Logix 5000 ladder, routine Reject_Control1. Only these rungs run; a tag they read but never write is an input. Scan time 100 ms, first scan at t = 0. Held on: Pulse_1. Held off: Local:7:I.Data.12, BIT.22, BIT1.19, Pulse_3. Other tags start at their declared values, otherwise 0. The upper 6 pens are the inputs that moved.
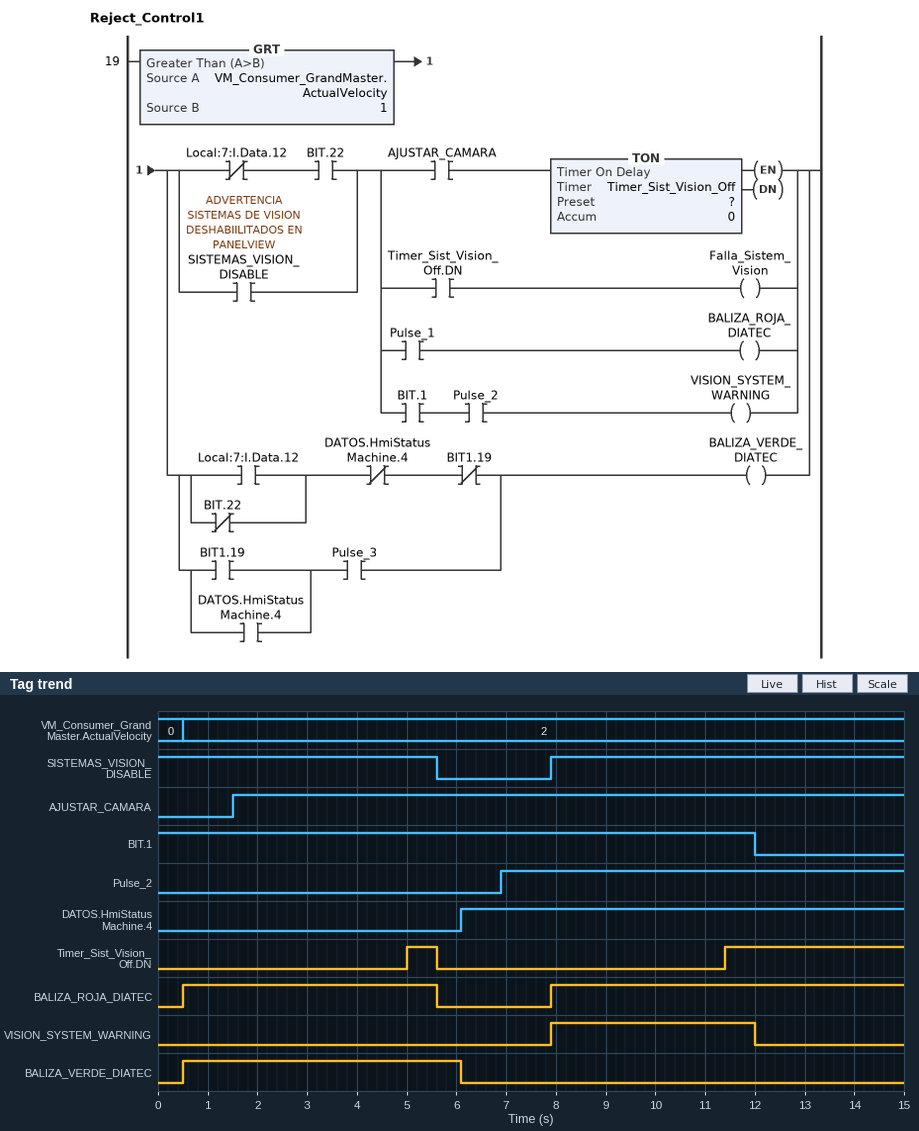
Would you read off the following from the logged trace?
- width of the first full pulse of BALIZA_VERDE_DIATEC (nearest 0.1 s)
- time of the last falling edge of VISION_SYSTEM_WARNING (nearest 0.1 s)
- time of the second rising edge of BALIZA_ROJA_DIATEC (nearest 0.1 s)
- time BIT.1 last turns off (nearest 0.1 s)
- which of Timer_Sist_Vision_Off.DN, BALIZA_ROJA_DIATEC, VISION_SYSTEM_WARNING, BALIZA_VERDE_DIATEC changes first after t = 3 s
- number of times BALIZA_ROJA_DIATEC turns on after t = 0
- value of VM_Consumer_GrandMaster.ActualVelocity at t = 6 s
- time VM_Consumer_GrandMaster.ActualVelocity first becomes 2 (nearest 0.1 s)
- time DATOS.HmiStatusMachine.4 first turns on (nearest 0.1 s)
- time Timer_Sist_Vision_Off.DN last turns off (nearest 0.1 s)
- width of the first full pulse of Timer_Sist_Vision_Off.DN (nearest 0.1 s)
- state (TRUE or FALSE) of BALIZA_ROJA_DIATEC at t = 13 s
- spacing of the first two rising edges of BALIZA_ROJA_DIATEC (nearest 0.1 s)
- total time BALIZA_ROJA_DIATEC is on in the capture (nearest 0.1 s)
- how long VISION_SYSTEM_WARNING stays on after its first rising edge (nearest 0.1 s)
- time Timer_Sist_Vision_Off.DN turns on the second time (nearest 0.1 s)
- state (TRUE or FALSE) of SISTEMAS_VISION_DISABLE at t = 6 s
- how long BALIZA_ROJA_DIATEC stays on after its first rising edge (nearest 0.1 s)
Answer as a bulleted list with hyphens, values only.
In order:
- 5.6 s
- 12.0 s
- 7.9 s
- 12.0 s
- Timer_Sist_Vision_Off.DN
- 2
- 2
- 0.5 s
- 6.1 s
- 5.6 s
- 0.6 s
- TRUE
- 7.4 s
- 12.2 s
- 4.1 s
- 11.4 s
- FALSE
- 5.1 s
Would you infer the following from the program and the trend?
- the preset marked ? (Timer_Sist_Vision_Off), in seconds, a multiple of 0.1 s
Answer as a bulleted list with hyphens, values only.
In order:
- 3.5 s
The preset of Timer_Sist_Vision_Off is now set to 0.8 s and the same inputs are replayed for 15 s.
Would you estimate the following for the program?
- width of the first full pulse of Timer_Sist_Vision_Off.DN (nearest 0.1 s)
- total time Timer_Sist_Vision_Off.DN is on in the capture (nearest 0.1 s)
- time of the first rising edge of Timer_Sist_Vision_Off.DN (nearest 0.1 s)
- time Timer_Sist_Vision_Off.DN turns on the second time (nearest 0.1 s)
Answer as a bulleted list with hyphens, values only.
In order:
- 3.3 s
- 9.6 s
- 2.3 s
- 8.7 s
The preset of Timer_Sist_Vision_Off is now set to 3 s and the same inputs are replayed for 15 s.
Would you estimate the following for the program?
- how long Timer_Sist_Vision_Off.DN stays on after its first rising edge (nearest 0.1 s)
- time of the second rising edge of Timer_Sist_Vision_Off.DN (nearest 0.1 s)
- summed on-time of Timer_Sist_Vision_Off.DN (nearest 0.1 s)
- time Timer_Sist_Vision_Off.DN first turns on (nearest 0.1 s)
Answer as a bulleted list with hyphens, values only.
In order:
- 1.1 s
- 10.9 s
- 5.2 s
- 4.5 s
